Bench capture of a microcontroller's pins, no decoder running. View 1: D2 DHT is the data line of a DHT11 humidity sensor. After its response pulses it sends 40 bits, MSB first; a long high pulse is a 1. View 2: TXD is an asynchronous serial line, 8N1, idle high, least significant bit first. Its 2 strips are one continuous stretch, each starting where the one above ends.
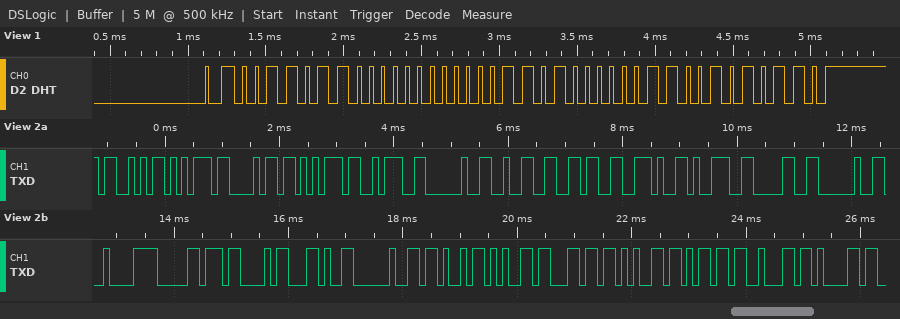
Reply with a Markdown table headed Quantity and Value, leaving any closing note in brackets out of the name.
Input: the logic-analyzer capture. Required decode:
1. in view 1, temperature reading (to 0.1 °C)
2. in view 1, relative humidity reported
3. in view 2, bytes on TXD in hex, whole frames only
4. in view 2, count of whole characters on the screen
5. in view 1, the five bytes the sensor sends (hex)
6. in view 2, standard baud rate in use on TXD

| Quantity | Value |
|---|---|
| in view 1, temperature reading | 26.6 °C |
| in view 1, relative humidity reported | 54 % |
| in view 2, bytes on TXD in hex, whole frames only | 0x53 0x75 0x68 0x75 0x3A 0x20 0x32 0x36 0x2E 0x39 0x30 0x20 0xC2 0xB0 0x43 0x2C 0x20 0x4B 0x65 0x6C 0x65 0x6D 0x62 0x61 |
| in view 2, count of whole characters on the screen | 24 |
| in view 1, the five bytes the sensor sends | 36 00 1A 06 56 |
| in view 2, standard baud rate in use on TXD | 9600 baud |
